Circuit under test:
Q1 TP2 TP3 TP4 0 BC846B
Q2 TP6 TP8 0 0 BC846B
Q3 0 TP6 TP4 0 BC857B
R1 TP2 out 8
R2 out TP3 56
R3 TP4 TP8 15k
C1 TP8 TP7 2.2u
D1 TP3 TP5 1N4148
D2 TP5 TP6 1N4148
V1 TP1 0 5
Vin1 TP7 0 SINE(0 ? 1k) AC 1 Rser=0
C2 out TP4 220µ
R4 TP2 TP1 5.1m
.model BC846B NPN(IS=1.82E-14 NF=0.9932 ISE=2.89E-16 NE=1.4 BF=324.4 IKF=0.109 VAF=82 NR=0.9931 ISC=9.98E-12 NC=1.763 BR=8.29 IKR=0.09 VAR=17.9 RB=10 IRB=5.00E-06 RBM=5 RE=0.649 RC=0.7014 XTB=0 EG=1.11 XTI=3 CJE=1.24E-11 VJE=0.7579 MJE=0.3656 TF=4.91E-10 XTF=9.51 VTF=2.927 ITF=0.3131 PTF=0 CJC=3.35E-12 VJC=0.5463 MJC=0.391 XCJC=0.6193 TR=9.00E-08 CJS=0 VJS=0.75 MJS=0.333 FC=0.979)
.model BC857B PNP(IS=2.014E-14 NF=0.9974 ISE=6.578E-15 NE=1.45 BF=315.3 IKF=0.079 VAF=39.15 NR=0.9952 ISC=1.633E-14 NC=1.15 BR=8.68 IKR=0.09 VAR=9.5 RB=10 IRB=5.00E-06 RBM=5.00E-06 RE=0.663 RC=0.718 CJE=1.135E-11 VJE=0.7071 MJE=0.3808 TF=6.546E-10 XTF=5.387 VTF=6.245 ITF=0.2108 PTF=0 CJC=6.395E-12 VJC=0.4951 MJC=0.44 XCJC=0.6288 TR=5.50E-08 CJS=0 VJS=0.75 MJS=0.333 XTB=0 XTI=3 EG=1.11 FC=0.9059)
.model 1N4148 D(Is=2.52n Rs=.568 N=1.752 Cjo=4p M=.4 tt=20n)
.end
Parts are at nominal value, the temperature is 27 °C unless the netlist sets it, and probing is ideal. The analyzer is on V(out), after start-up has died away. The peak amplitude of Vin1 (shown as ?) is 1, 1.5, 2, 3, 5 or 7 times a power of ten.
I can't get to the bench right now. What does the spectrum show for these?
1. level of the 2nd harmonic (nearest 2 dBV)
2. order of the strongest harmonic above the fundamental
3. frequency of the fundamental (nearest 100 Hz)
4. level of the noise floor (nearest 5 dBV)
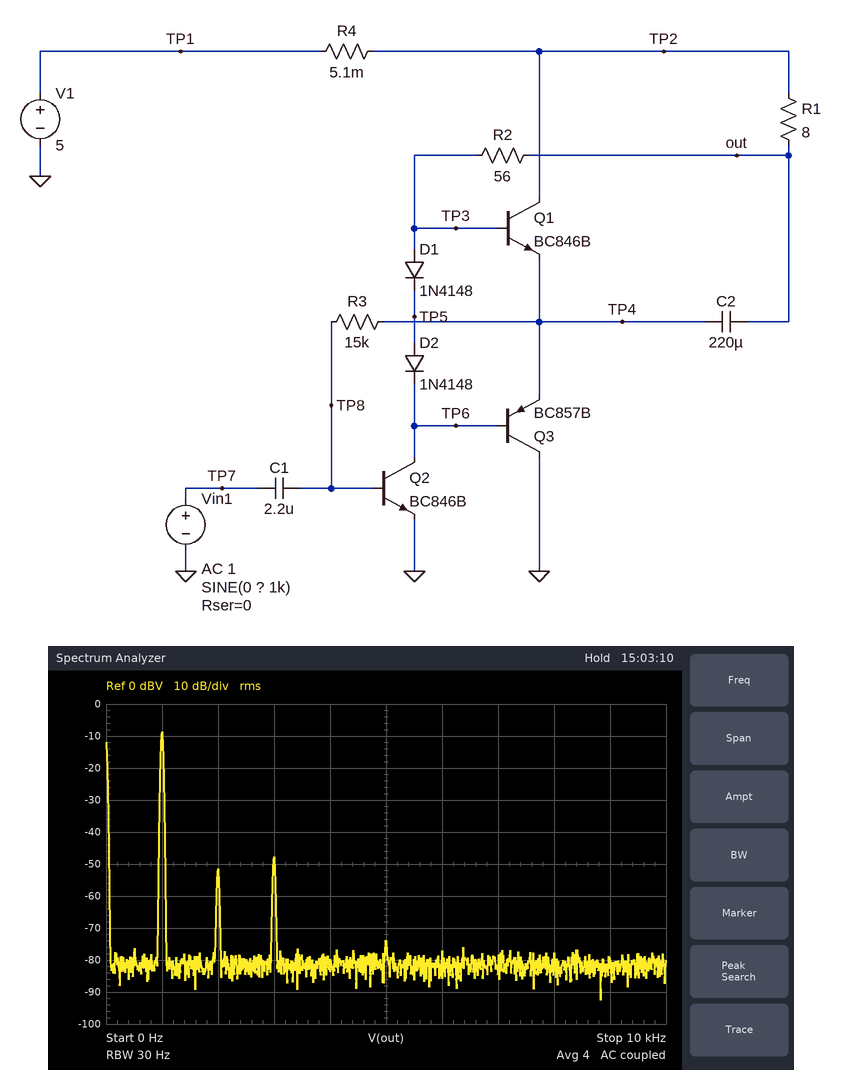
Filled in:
-52 dBV
3
1.0 kHz
-80 dBV
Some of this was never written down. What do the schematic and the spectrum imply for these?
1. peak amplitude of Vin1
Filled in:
5 mV
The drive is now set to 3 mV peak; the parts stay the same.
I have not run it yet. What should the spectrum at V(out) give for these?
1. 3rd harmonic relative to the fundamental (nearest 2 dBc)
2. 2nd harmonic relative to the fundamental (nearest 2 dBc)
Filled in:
-48 dBc
-48 dBc
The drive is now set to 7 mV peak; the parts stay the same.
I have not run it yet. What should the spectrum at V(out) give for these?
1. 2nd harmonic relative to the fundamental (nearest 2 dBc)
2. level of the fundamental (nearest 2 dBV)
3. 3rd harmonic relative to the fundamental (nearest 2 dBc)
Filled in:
-40 dBc
-6 dBV
-34 dBc
